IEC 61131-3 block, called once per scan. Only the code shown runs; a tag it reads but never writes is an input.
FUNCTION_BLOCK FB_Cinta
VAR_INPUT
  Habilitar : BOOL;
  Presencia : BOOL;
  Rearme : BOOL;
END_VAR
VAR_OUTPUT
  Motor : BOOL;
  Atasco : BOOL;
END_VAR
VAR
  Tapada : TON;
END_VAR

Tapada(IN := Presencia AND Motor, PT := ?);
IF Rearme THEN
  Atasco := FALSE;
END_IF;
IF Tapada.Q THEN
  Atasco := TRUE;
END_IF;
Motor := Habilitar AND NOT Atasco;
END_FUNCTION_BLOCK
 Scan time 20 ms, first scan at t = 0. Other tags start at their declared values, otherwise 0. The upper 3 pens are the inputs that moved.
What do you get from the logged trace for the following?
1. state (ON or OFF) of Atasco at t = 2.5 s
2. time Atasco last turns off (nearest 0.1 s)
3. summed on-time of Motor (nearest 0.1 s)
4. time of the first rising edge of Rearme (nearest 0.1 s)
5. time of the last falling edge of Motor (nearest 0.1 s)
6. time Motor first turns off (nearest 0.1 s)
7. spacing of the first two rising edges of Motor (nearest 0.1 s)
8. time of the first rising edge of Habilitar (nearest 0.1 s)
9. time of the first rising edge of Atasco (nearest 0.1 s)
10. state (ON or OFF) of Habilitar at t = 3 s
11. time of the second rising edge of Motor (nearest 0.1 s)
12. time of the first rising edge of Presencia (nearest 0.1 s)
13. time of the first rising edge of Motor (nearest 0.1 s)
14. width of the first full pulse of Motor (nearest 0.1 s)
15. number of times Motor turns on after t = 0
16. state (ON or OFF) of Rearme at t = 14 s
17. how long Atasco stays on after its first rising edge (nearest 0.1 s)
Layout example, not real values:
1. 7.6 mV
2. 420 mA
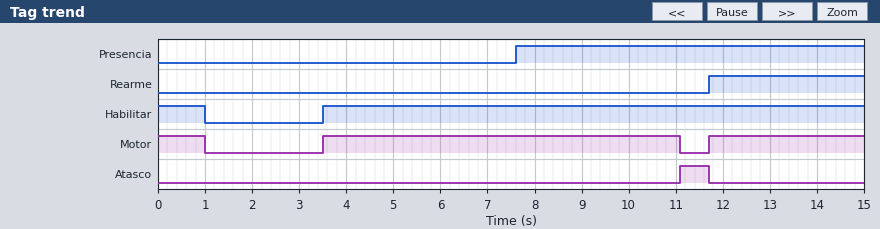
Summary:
1. OFF
2. 11.7 s
3. 11.9 s
4. 11.7 s
5. 11.1 s
6. 1.0 s
7. 8.2 s
8. 3.5 s
9. 11.1 s
10. OFF
11. 11.7 s
12. 7.6 s
13. 3.5 s
14. 7.6 s
15. 2
16. ON
17. 0.6 s
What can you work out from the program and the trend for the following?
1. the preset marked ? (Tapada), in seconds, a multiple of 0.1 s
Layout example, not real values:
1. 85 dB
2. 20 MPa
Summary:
1. 3.5 s
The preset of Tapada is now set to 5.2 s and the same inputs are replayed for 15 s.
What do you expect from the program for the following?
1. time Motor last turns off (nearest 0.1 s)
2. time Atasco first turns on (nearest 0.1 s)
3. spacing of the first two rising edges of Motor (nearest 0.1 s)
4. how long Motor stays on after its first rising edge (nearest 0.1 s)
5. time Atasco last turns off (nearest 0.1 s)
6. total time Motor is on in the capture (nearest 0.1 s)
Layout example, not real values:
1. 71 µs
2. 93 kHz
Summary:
1. 12.8 s
2. 12.8 s
3. 9.3 s
4. 9.3 s
5. 12.8 s
6. 12.5 s
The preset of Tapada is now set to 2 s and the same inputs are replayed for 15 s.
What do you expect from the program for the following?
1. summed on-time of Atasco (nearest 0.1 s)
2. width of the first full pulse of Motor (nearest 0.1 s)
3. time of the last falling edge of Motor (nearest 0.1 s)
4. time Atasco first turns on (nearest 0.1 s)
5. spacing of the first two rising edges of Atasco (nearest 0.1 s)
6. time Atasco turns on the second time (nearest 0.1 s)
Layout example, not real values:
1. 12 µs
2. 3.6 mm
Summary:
1. 2.1 s
2. 6.1 s
3. 13.7 s
4. 9.6 s
5. 4.1 s
6. 13.7 s
